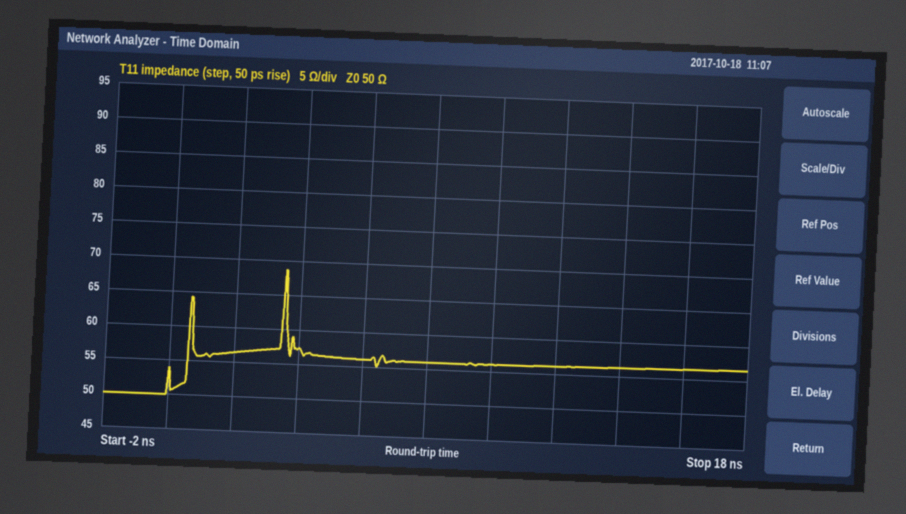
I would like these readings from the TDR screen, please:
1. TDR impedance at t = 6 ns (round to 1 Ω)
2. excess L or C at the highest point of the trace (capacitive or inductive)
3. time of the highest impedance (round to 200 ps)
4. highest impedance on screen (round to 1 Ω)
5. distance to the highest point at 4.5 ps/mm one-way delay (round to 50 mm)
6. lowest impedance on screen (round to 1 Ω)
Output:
56 Ω
inductive
3.6 ns
69 Ω
400 mm
50 Ω
